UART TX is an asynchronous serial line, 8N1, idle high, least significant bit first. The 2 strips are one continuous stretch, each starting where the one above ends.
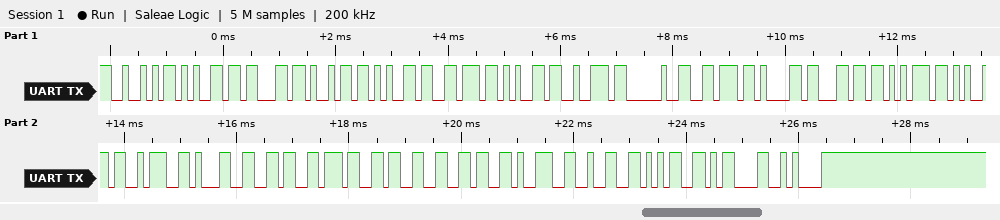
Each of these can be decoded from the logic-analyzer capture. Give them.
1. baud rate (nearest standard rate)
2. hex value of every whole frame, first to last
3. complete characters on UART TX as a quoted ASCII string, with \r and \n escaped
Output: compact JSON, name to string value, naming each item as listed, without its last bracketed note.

{"baud rate": "9600 baud", "hex value of every whole frame, first to last": "0x52 0x65 0x63 0x69 0x65 0x76 0x65 0x72 0x20 0x76 0x61 0x6C 0x75 0x65 0x3A 0x31 0x36 0x37 0x33 0x36 0x39 0x32 0x35 0x0D 0x0A", "complete characters on UART TX as a quoted ASCII string, with \\r and \\n escaped": "\"Reciever value:16736925\\r\\n\""}
